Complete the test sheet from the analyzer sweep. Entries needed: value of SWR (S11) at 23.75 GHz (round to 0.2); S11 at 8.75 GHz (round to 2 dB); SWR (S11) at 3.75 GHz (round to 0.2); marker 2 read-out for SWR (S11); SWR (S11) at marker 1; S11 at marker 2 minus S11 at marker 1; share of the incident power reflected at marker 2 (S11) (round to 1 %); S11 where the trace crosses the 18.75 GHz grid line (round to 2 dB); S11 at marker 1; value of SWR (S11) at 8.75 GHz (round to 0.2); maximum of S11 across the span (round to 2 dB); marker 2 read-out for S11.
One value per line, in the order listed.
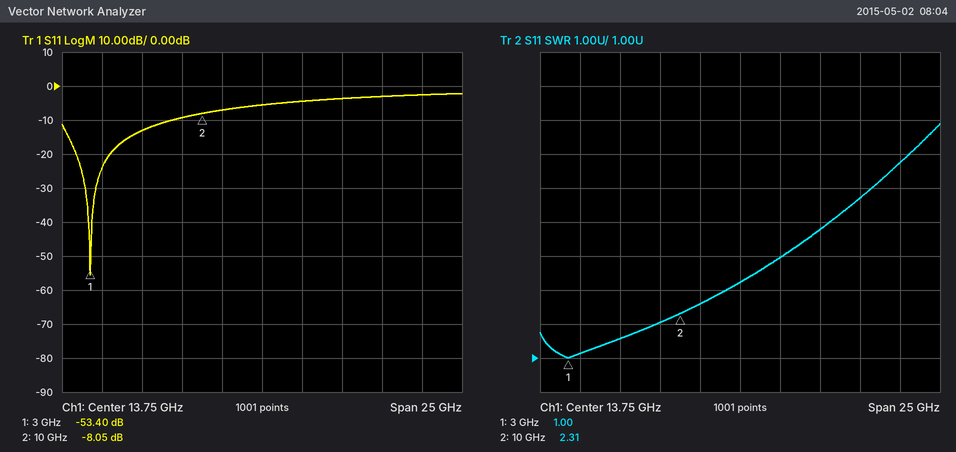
6.8
-10 dB
1.2
2.31
1.00
45.35 dB
16 %
-4 dB
-53.40 dB
2.0
-2 dB
-8.05 dB
